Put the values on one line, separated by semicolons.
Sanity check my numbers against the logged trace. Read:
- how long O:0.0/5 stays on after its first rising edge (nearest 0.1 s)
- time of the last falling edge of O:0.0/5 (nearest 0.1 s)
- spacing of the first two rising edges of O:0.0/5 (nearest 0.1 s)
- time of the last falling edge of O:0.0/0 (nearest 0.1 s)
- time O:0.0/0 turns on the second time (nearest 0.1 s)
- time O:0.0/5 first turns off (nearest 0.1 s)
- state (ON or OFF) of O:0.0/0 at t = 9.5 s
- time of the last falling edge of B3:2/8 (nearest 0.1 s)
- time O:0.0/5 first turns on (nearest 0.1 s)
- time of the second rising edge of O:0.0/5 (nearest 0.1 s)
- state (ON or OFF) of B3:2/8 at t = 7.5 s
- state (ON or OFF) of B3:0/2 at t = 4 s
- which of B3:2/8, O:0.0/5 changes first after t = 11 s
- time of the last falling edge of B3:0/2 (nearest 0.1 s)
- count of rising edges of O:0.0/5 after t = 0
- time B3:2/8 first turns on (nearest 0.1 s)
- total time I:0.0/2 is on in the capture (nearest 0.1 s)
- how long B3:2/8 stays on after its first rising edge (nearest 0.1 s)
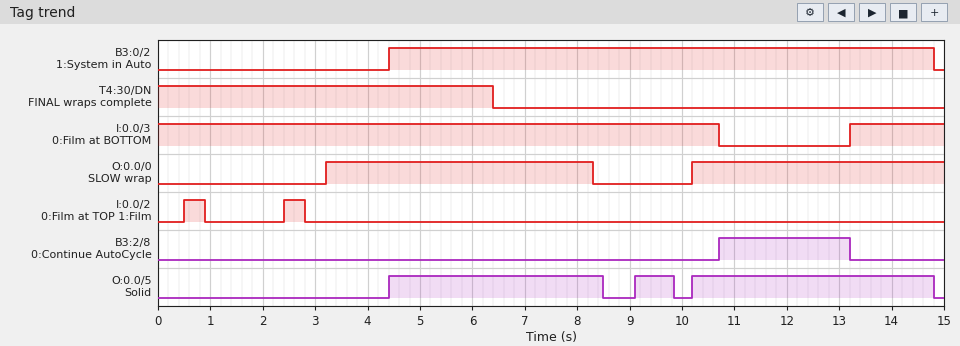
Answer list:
4.1 s; 14.8 s; 4.7 s; 8.3 s; 10.2 s; 8.5 s; OFF; 13.2 s; 4.4 s; 9.1 s; OFF; OFF; B3:2/8; 14.8 s; 3; 10.7 s; 0.8 s; 2.5 s
